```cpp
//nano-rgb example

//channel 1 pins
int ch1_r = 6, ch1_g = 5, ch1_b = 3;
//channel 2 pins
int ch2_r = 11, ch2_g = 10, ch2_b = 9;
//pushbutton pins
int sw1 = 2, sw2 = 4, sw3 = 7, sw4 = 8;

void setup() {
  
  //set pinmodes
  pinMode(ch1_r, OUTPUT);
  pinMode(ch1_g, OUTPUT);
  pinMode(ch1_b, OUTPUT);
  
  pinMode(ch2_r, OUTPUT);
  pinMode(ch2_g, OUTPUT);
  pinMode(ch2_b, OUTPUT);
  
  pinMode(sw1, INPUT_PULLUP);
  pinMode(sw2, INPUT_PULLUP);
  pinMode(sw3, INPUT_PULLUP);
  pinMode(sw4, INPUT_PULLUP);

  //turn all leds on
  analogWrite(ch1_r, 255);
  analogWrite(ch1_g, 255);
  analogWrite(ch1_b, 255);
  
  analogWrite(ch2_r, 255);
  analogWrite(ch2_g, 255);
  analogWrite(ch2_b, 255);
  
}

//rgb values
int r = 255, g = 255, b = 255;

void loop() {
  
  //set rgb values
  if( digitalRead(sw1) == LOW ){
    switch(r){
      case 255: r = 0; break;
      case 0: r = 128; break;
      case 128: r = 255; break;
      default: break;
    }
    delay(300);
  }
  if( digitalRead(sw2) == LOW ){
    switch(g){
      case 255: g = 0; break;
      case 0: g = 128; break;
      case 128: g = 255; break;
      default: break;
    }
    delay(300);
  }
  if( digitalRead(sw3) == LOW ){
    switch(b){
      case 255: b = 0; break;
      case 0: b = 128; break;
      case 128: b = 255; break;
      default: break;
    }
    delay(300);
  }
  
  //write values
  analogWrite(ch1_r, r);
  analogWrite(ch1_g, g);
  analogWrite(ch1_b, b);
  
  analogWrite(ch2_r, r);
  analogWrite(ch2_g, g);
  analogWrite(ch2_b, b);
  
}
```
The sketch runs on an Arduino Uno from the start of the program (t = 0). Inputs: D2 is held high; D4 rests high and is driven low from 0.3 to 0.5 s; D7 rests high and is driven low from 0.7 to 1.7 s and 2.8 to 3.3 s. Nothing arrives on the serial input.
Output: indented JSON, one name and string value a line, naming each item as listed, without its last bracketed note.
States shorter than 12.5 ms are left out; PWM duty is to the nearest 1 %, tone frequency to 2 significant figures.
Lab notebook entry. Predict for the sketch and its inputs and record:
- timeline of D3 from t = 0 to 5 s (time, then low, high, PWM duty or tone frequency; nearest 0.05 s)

{
  "timeline of D3 from t = 0 to 5 s": "0 s high; 1 s low; 1.3 s PWM 50 %; 1.6 s high; 1.9 s low; 3.1 s PWM 50 %; 3.4 s high"
}
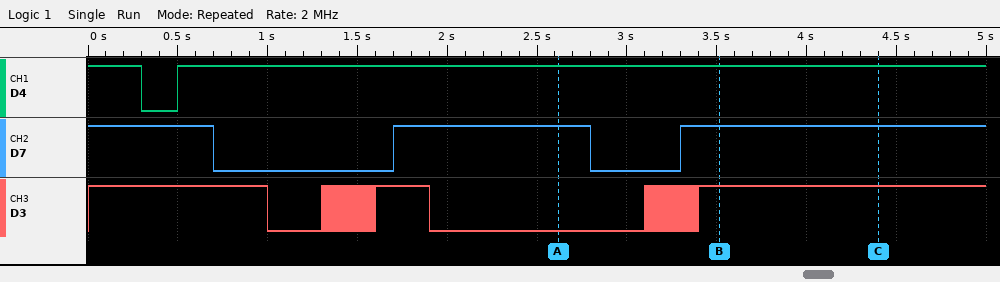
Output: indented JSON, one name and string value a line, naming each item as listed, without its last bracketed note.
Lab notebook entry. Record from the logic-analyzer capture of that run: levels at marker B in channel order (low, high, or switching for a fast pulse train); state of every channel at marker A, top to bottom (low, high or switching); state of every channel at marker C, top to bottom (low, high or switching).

{
  "levels at marker B in channel order": "D4 high, D7 high, D3 high",
  "state of every channel at marker A, top to bottom": "D4 high, D7 high, D3 low",
  "state of every channel at marker C, top to bottom": "D4 high, D7 high, D3 high"
}
